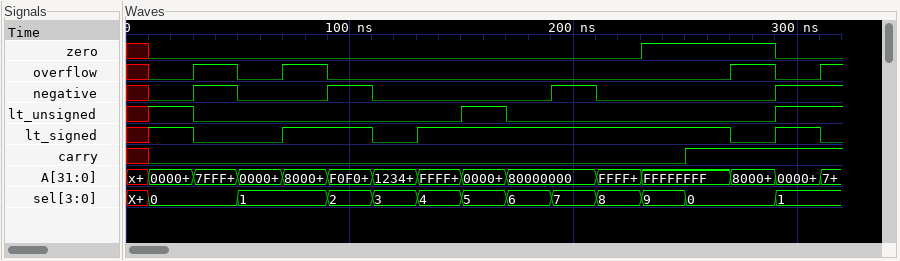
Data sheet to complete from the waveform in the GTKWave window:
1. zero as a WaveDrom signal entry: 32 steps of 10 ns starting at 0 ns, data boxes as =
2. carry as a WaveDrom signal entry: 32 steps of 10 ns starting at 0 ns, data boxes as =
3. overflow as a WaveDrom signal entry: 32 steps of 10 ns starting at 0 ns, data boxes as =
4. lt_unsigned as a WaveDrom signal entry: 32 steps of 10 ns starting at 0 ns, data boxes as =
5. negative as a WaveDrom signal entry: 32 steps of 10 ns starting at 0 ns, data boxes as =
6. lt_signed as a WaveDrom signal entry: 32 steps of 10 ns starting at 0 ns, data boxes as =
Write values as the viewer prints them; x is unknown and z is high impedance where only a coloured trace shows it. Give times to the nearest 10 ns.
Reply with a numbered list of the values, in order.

1. {name: 'zero', wave: 'x0.....................1.....0..'}
2. {name: 'carry', wave: 'x0.......................1......'}
3. {name: 'overflow', wave: 'x0.1.0.1.0.................1.0.1'}
4. {name: 'lt_unsigned', wave: 'x1.0...........1.0...........1..'}
5. {name: 'negative', wave: 'x0.1.0...1.0.......1.0.......1..'}
6. {name: 'lt_signed', wave: 'x1.0...1...0.1.............0.1.0'}
